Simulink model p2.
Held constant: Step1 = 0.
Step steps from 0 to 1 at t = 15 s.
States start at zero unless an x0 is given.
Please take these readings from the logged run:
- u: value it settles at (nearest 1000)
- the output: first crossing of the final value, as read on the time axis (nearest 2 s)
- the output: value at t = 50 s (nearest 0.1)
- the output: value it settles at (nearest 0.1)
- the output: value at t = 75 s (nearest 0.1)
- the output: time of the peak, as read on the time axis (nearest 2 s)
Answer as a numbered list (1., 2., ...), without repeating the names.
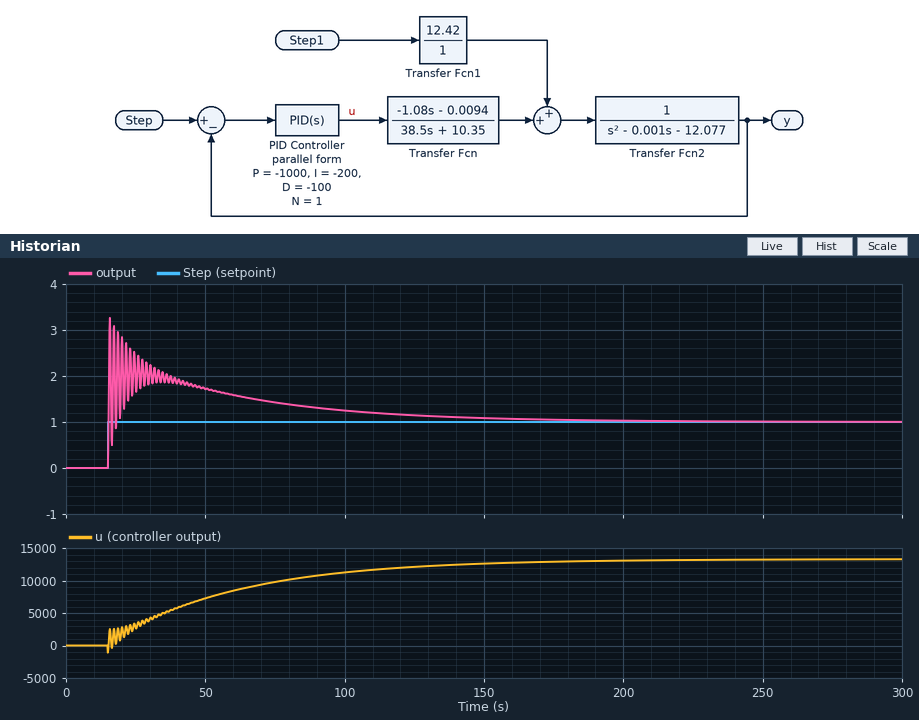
1. 13000
2. 16 s
3. 1.7
4. 1.0
5. 1.4
6. 16 s
